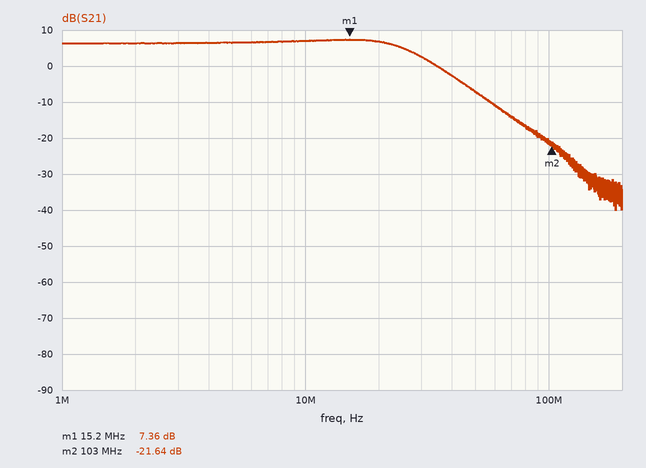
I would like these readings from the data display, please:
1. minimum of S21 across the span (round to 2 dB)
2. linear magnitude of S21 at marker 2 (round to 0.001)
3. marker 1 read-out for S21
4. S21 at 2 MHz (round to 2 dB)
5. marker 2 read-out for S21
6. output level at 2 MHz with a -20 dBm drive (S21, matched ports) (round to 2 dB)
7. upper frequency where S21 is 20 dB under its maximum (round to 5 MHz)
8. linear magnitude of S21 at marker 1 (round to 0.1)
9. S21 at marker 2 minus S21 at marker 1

-40 dB
0.083
7.36 dB
6 dB
-21.64 dB
-14 dBm
65 MHz
2.3
-29.00 dB
